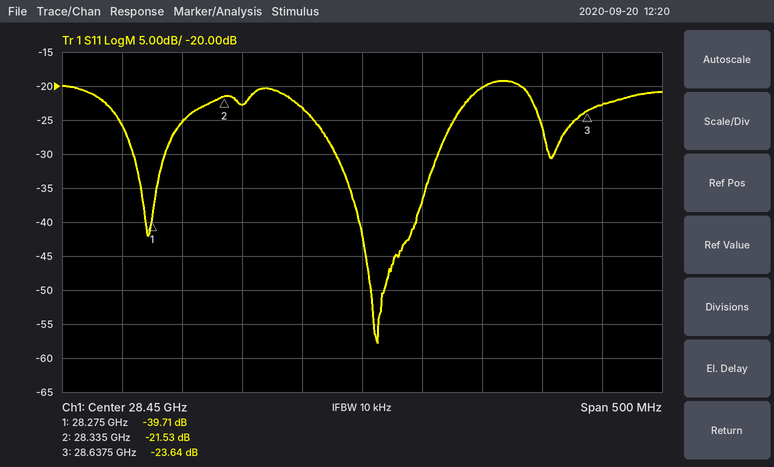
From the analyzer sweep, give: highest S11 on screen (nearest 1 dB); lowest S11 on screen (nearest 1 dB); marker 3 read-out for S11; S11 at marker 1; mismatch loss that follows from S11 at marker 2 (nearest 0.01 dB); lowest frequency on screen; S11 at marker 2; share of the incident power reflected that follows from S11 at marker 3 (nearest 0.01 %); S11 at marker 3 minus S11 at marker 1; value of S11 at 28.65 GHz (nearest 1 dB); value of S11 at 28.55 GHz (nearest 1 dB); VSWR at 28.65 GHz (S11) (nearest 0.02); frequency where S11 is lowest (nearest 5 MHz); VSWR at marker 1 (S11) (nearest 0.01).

-19 dB
-58 dB
-23.64 dB
-39.71 dB
0.03 dB
28.2 GHz
-21.53 dB
0.43 %
16.07 dB
-23 dB
-20 dB
1.16
28.465 GHz
1.02
